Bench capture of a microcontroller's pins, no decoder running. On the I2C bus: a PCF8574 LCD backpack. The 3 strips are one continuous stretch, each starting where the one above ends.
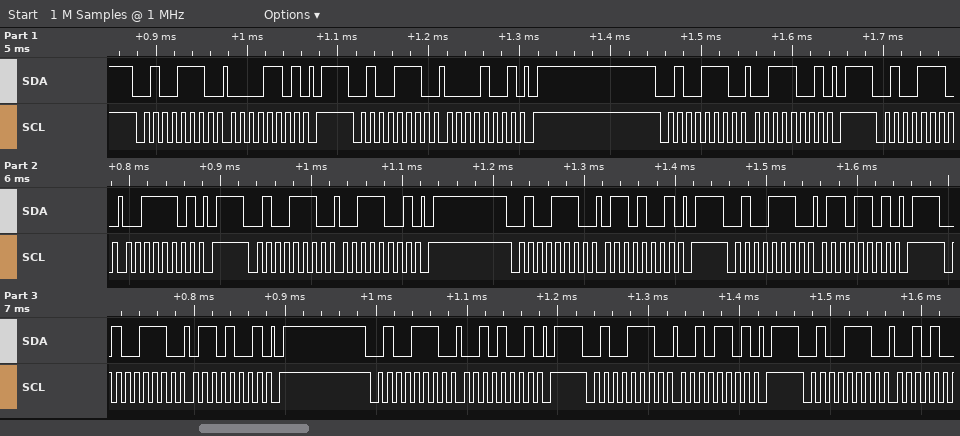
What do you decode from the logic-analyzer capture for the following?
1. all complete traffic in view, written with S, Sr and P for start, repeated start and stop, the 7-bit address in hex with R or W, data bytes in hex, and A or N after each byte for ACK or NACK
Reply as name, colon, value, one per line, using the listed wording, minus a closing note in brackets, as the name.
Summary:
all complete traffic in view, written with S, Sr and P for start, repeated start and stop, the 7-bit address in hex with R or W, data bytes in hex, and A or N after each byte for ACK or NACK: S 27W A 0D A P S 27W A 09 A P S 27W A 39 A P S 27W A 3D A P S 27W A 39 A P S 27W A 69 A P S 27W A 6D A P S 27W A 69 A P S 27W A 29 A P S 27W A 2D A P S 27W A
